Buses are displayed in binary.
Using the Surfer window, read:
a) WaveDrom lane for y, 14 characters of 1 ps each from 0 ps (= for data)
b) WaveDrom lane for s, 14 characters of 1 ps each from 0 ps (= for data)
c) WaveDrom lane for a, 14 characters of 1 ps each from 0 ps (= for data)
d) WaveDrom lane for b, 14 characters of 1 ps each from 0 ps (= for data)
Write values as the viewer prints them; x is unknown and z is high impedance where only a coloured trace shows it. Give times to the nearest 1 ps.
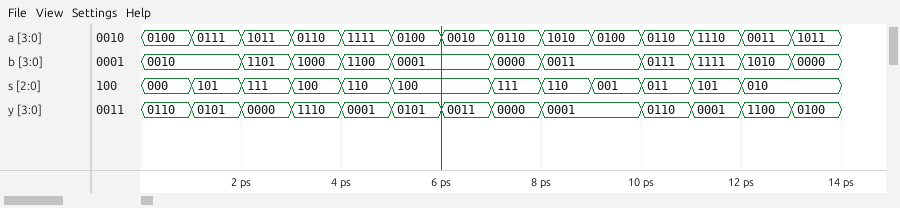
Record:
{name: 'y', wave: '=========.====', data: '0110 0101 0000 1110 0001 0101 0011 0000 0001 0110 0001 1100 0100'}
{name: 's', wave: '======.======.', data: '000 101 111 100 110 100 111 110 001 011 101 010'}
{name: 'a', wave: '==============', data: '0100 0111 1011 0110 1111 0100 0010 0110 1010 0100 0110 1110 0011 1011'}
{name: 'b', wave: '=.====.==.====', data: '0010 1101 1000 1100 0001 0000 0011 0111 1111 1010 0000'}
